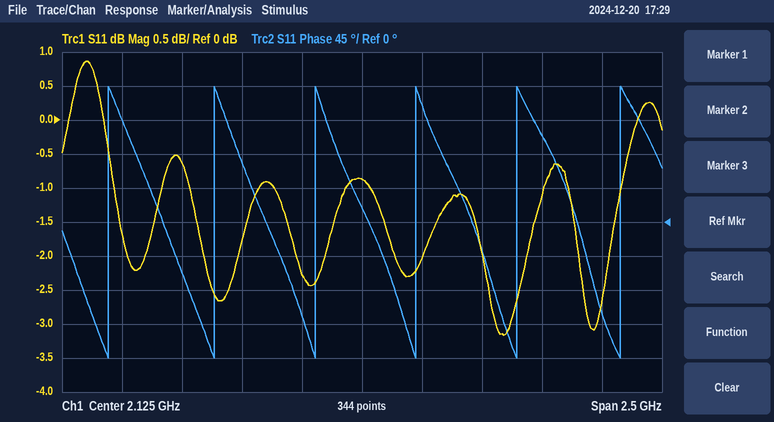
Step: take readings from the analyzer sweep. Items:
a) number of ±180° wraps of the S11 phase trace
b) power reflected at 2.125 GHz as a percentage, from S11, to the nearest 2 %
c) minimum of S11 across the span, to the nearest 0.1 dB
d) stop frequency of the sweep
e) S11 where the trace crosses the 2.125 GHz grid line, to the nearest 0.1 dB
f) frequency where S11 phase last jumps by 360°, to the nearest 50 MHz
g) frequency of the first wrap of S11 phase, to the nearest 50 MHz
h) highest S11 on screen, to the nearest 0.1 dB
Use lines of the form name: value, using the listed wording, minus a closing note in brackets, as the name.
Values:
number of ±180° wraps of the S11 phase trace: 6
power reflected at 2.125 GHz as a percentage, from S11, to the nearest 2 %: 82 %
minimum of S11 across the span, to the nearest 0.1 dB: -3.2 dB
stop frequency of the sweep: 3.375 GHz
S11 where the trace crosses the 2.125 GHz grid line, to the nearest 0.1 dB: -0.9 dB
frequency where S11 phase last jumps by 360°, to the nearest 50 MHz: 3.20 GHz
frequency of the first wrap of S11 phase, to the nearest 50 MHz: 1.05 GHz
highest S11 on screen, to the nearest 0.1 dB: 0.9 dB
